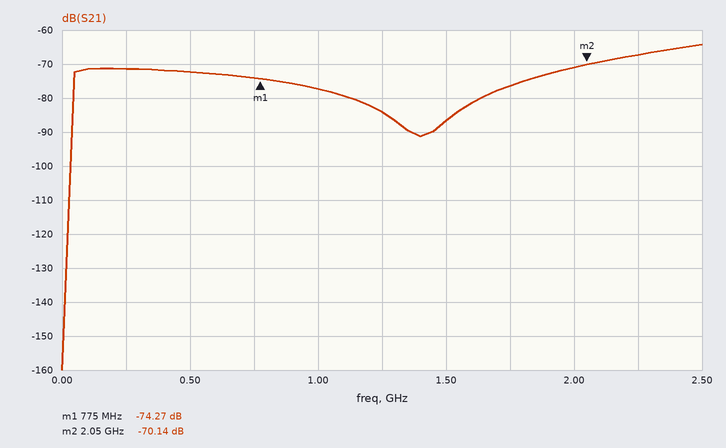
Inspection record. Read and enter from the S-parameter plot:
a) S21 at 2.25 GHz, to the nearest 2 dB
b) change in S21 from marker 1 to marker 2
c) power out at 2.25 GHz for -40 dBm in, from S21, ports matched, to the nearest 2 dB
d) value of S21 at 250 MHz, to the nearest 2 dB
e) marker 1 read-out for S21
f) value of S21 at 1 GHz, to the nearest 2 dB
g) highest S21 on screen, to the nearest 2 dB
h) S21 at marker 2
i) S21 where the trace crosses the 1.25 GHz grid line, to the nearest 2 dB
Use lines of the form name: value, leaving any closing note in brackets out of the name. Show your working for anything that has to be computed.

S21 at 2.25 GHz, to the nearest 2 dB: -68 dB
change in S21 from marker 1 to marker 2: -70.14 − (-74.27) = 4.13 dB
power out at 2.25 GHz for -40 dBm in, from S21, ports matched, to the nearest 2 dB: -40 dBm + (-68 dB) = -108 dBm
value of S21 at 250 MHz, to the nearest 2 dB: -72 dB
marker 1 read-out for S21: -74.27 dB
value of S21 at 1 GHz, to the nearest 2 dB: -78 dB
highest S21 on screen, to the nearest 2 dB: -64 dB
S21 at marker 2: -70.14 dB
S21 where the trace crosses the 1.25 GHz grid line, to the nearest 2 dB: -84 dB
